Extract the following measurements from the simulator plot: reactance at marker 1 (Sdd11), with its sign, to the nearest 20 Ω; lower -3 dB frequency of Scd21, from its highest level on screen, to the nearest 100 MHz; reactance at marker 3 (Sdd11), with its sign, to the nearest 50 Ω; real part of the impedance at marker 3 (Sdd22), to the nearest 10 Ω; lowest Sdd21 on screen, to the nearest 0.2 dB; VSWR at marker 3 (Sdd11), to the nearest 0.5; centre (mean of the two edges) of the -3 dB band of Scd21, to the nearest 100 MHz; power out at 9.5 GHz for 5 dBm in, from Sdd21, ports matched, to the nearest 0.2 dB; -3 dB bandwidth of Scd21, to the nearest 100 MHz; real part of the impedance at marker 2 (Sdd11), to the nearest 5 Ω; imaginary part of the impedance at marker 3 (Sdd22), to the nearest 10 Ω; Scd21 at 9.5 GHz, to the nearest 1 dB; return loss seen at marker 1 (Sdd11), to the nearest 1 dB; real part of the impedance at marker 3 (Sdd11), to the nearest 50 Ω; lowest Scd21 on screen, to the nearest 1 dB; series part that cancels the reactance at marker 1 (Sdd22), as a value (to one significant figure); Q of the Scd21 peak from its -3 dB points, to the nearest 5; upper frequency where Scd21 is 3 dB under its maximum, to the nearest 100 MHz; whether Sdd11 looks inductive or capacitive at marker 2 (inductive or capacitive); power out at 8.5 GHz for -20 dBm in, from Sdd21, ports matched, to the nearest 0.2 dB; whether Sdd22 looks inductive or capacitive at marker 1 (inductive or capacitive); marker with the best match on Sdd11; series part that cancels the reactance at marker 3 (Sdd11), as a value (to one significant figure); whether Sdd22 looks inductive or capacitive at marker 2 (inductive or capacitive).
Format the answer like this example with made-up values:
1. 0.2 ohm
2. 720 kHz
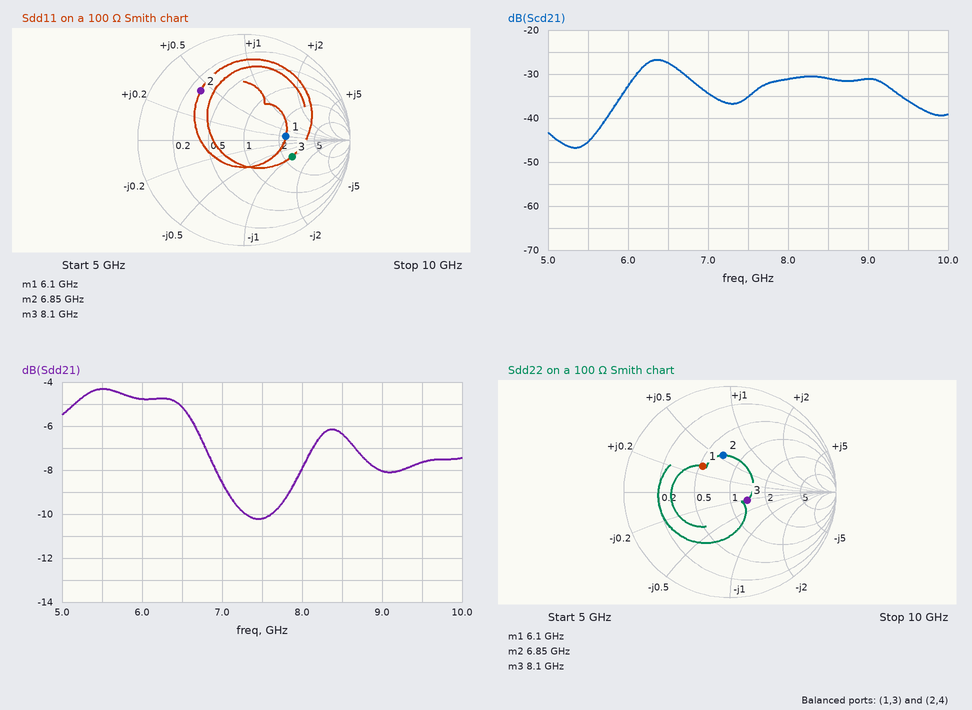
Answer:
1. +20 Ω
2. 6.1 GHz
3. -100 Ω
4. 140 Ω
5. -10.2 dB
6. 3.0
7. 6.4 GHz
8. -2.6 dBm
9. 600 MHz
10. 30 Ω
11. -20 Ω
12. -36 dB
13. 8 dB
14. 250 Ω
15. -47 dB
16. 900 fF
17. 10
18. 6.7 GHz
19. inductive
20. -26.4 dBm
21. inductive
22. marker 1
23. 2 nH
24. inductive
